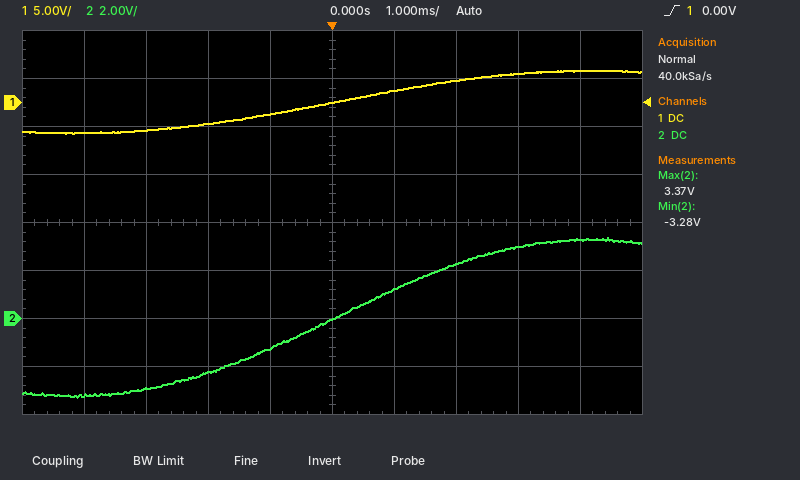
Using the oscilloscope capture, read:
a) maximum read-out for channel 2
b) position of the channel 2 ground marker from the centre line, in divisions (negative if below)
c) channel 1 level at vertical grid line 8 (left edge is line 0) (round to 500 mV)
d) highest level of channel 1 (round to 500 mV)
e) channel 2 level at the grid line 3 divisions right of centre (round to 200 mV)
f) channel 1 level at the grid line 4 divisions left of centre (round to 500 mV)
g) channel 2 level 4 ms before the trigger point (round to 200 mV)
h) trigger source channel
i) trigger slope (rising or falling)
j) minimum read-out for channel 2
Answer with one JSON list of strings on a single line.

["3.37 V", "-2.0 div", "3.0 V", "3.5 V", "3.0 V", "-3.0 V", "-3.2 V", "channel 1", "rising", "-3.28 V"]
